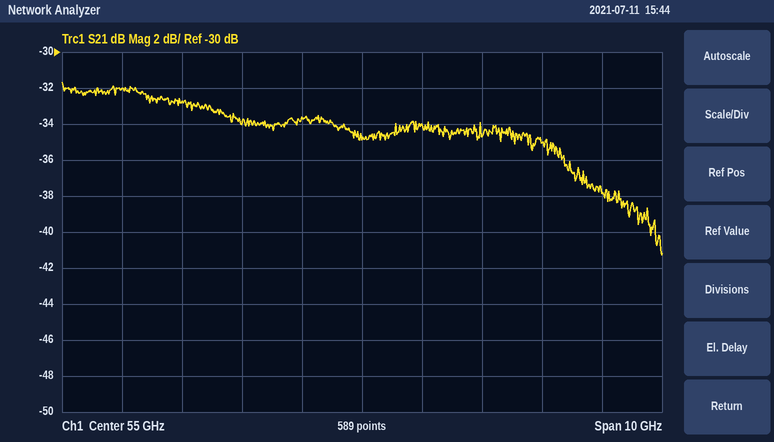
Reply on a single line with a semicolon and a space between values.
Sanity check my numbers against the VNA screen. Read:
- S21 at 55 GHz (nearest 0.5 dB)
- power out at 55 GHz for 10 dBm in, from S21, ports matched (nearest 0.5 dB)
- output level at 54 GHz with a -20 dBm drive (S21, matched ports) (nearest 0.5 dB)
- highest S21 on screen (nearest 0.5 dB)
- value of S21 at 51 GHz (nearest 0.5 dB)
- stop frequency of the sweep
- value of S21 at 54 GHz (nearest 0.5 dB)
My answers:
-35.0 dB; -25.0 dBm; -53.5 dBm; -31.5 dB; -32.0 dB; 60 GHz; -33.5 dB
